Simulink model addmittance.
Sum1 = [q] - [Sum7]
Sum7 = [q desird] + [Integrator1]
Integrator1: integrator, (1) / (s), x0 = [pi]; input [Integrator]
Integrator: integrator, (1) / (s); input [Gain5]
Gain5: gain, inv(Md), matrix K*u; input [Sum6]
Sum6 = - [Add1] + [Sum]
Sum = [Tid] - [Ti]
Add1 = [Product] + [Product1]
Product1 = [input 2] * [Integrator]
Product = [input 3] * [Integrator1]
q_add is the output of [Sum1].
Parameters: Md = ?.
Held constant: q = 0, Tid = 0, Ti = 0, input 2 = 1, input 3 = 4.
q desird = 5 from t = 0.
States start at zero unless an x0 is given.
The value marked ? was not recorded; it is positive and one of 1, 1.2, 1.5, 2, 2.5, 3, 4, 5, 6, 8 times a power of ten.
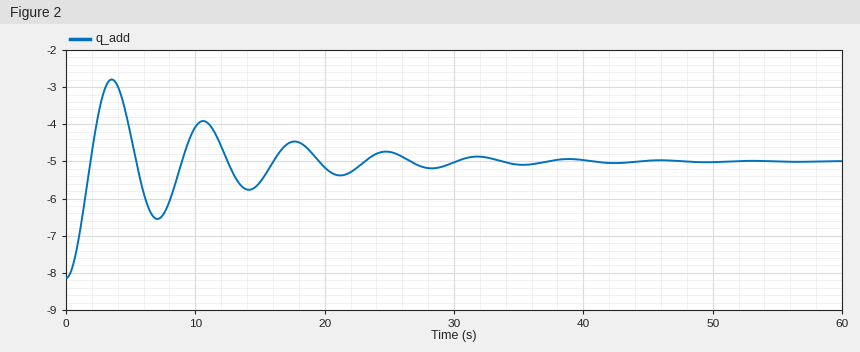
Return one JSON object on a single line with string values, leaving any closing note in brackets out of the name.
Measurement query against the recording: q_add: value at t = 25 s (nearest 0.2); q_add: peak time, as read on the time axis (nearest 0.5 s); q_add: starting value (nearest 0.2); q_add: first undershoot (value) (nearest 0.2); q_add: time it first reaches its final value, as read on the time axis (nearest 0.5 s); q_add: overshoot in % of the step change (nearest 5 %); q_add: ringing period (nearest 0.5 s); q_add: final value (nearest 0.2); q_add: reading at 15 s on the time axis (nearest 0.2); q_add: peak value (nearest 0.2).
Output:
{"q_add: value at t = 25 s": "-4.8", "q_add: peak time, as read on the time axis": "3.5 s", "q_add: starting value": "-8.2", "q_add: first undershoot (value)": "-6.6", "q_add: time it first reaches its final value, as read on the time axis": "2.0 s", "q_add: overshoot in % of the step change": "70 %", "q_add: ringing period": "7.0 s", "q_add: final value": "-5.0", "q_add: reading at 15 s on the time axis": "-5.6", "q_add: peak value": "-2.8"}
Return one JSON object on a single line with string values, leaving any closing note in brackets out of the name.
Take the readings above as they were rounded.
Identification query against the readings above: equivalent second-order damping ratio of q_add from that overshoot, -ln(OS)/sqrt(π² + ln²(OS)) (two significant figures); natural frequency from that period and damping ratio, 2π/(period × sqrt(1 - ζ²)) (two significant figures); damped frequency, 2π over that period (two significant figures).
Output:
{"equivalent second-order damping ratio of q_add from that overshoot, -ln(OS)/sqrt(π² + ln²(OS))": "0.11", "natural frequency from that period and damping ratio, 2π/(period × sqrt(1 - ζ²))": "0.90 rad/s", "damped frequency, 2π over that period": "0.90 rad/s"}
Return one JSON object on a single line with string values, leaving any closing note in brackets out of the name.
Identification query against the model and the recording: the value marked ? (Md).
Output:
{"the value marked ?": "5"}
